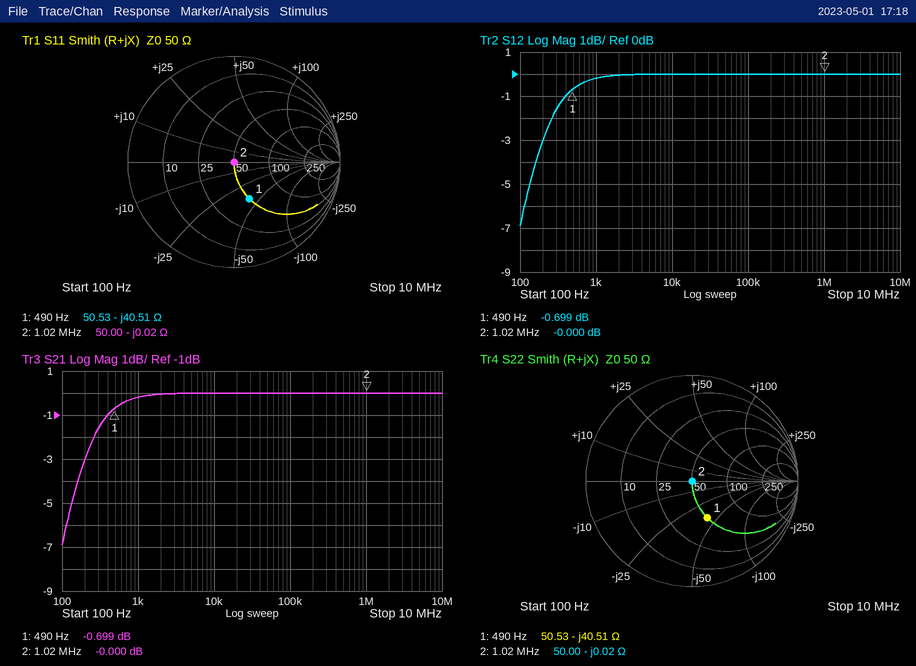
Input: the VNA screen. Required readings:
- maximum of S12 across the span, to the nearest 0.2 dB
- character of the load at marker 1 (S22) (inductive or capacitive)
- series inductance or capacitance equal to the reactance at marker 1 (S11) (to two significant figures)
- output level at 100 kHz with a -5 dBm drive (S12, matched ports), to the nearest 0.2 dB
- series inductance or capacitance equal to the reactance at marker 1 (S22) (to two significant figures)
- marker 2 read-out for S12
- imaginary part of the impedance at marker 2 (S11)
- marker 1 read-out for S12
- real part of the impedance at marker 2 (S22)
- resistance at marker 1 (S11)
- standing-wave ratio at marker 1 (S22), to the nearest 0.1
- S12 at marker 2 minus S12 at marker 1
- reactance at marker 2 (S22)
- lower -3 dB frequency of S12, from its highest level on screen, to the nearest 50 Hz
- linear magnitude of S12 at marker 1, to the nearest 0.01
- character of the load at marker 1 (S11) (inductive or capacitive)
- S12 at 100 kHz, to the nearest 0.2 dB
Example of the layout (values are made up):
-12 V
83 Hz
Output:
0.0 dB
capacitive
8.0 µF
-5.0 dBm
8.0 µF
-0.000 dB
-0.02 Ω
-0.699 dB
50.00 Ω
50.53 Ω
2.2
0.699 dB
-0.02 Ω
200 Hz
0.92
capacitive
0.0 dB
